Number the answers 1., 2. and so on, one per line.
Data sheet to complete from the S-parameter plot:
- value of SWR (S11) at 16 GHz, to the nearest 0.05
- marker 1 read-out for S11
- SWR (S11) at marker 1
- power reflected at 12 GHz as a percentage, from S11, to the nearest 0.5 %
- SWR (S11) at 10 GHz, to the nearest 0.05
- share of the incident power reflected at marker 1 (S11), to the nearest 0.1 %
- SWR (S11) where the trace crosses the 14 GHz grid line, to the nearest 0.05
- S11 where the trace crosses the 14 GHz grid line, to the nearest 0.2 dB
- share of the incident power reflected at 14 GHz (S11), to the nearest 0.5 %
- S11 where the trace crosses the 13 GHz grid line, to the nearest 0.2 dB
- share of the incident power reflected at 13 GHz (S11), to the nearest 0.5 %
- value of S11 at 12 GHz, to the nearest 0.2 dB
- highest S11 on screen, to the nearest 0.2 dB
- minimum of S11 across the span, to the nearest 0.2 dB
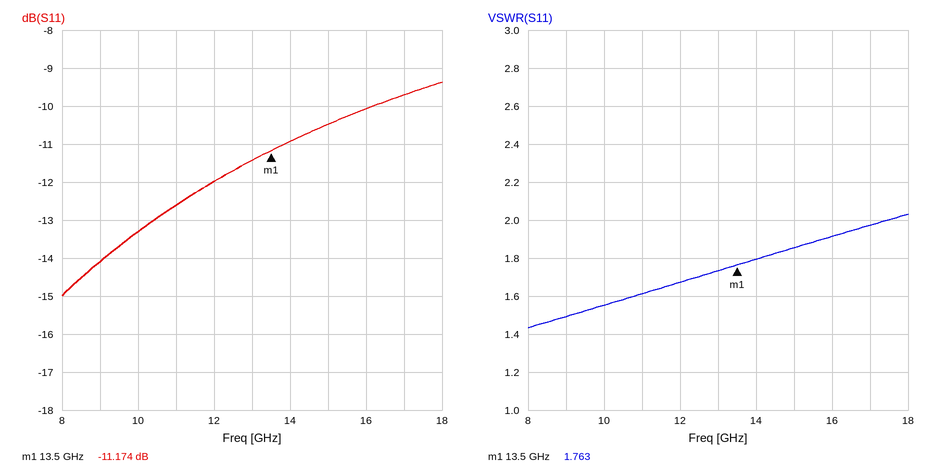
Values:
1. 1.90
2. -11.174 dB
3. 1.763
4. 6.5 %
5. 1.55
6. 7.6 %
7. 1.80
8. -11.0 dB
9. 8.0 %
10. -11.4 dB
11. 7.0 %
12. -12.0 dB
13. -9.4 dB
14. -15.0 dB
